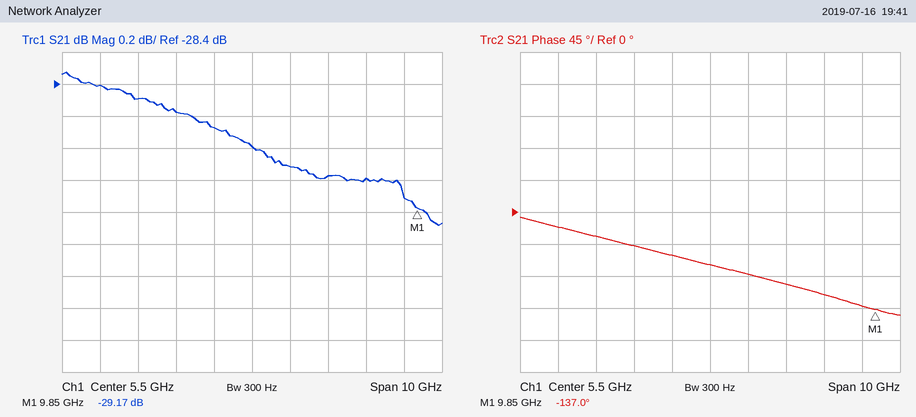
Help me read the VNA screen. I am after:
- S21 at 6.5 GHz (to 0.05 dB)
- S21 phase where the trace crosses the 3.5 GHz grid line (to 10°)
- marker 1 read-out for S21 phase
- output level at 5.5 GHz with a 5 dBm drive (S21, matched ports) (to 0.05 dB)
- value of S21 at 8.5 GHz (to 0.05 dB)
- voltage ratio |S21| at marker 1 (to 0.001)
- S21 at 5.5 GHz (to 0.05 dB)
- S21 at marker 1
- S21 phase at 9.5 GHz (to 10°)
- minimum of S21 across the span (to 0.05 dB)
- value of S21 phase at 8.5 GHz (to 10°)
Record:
-28.90 dB
-50°
-137.0°
-23.80 dBm
-29.00 dB
0.035
-28.80 dB
-29.17 dB
-130°
-29.30 dB
-120°
